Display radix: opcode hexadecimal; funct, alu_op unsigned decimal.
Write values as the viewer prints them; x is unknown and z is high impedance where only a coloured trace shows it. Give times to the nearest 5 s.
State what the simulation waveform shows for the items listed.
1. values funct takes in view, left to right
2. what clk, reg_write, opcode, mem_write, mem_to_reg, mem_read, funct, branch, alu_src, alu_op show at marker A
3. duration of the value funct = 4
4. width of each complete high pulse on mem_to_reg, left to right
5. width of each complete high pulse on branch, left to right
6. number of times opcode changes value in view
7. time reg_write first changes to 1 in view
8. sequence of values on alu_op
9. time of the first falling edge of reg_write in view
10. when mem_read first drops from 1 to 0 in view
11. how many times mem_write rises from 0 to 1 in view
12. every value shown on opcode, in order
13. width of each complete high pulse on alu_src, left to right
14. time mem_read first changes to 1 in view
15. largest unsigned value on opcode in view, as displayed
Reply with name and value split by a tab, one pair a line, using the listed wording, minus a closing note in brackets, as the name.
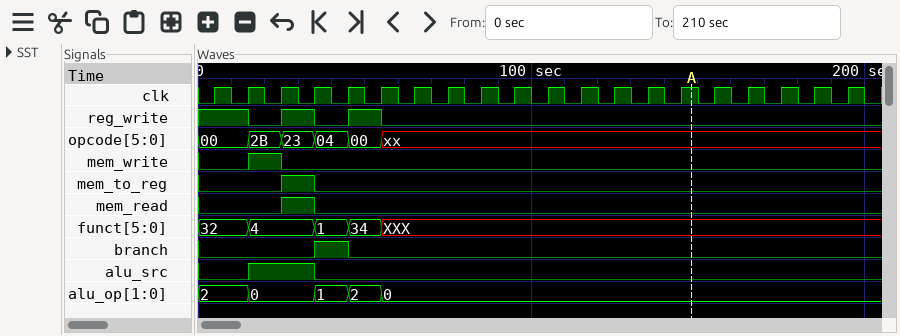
values funct takes in view, left to right	32, 4, 1, 34, XXX
what clk, reg_write, opcode, mem_write, mem_to_reg, mem_read, funct, branch, alu_src, alu_op show at marker A	clk=1, reg_write=0, opcode=xx, mem_write=0, mem_to_reg=0, mem_read=0, funct=XXX, branch=0, alu_src=0, alu_op=0
duration of the value funct = 4	20 s
width of each complete high pulse on mem_to_reg, left to right	10 s
width of each complete high pulse on branch, left to right	10 s
number of times opcode changes value in view	5
time reg_write first changes to 1 in view	25 s
sequence of values on alu_op	2, 0, 1, 2, 0
time of the first falling edge of reg_write in view	15 s
when mem_read first drops from 1 to 0 in view	35 s
how many times mem_write rises from 0 to 1 in view	1
every value shown on opcode, in order	00, 2B, 23, 04, 00, xx
width of each complete high pulse on alu_src, left to right	20 s
time mem_read first changes to 1 in view	25 s
largest unsigned value on opcode in view, as displayed	2B
